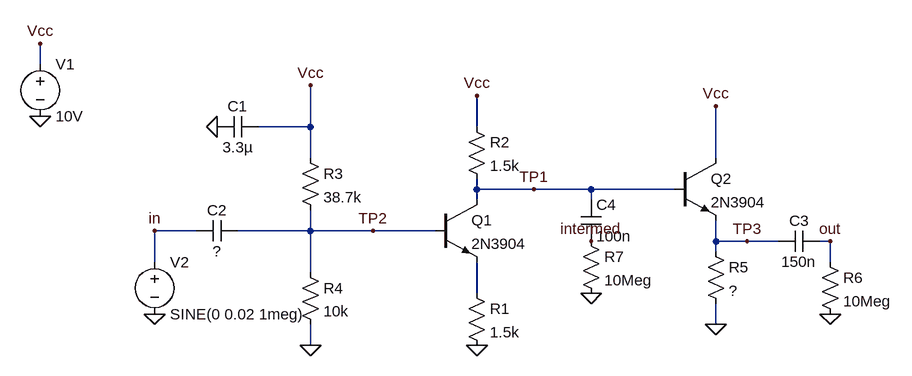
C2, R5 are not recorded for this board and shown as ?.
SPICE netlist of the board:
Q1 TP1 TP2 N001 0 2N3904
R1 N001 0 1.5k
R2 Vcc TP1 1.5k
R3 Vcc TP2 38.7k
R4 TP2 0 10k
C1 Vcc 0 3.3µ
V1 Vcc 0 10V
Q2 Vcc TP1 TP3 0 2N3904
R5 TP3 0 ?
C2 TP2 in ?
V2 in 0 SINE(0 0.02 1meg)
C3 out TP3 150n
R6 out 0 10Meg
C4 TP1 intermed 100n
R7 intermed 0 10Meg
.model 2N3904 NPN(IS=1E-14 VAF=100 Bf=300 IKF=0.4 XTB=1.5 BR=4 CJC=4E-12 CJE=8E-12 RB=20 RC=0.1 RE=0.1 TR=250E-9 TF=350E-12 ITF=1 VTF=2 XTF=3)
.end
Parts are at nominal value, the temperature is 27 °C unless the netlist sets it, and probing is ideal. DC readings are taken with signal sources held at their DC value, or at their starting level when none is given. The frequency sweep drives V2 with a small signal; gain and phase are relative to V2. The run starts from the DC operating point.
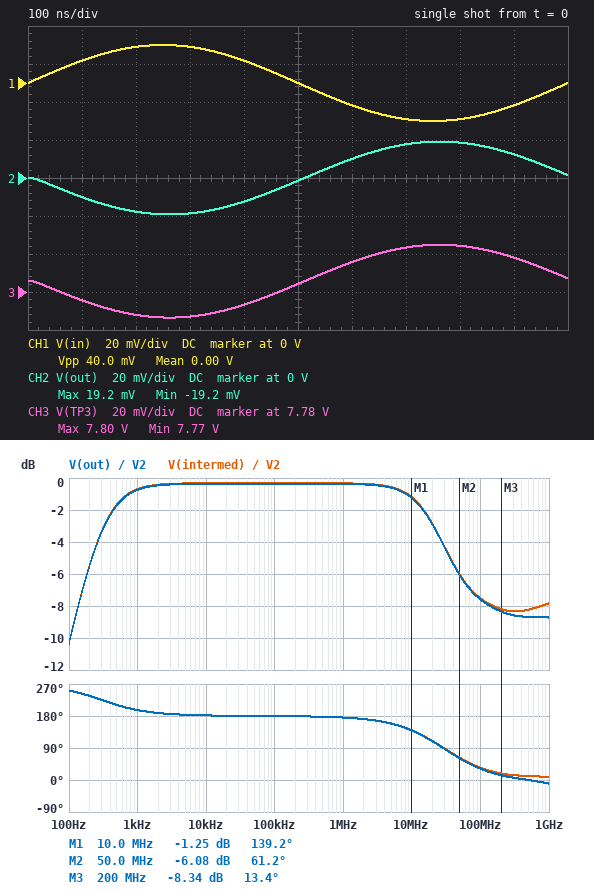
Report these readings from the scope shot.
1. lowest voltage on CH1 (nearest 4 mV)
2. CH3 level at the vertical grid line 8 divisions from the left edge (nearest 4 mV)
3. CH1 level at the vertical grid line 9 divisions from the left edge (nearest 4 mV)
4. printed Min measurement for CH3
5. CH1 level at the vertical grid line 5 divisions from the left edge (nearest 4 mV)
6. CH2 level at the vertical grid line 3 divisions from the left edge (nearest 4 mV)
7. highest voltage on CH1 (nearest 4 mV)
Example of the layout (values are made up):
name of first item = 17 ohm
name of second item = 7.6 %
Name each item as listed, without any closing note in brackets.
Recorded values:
lowest voltage on CH1 = -20 mV
CH3 level at the vertical grid line 8 divisions from the left edge = 7.804 V
CH1 level at the vertical grid line 9 divisions from the left edge = -12 mV
printed Min measurement for CH3 = 7.77 V
CH1 level at the vertical grid line 5 divisions from the left edge = 0 V
CH2 level at the vertical grid line 3 divisions from the left edge = -20 mV
highest voltage on CH1 = 20 mV
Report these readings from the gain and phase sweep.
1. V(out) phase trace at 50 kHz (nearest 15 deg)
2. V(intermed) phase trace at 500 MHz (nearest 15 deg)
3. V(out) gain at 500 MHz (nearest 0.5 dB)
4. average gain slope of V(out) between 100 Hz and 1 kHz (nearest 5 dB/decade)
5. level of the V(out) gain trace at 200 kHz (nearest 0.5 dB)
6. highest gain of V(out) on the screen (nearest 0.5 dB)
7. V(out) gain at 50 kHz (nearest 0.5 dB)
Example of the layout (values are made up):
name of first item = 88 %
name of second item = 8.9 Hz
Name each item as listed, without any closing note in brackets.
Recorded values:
V(out) phase trace at 50 kHz = 180 deg
V(intermed) phase trace at 500 MHz = 15 deg
V(out) gain at 500 MHz = -8.5 dB
average gain slope of V(out) between 100 Hz and 1 kHz = 10 dB/decade
level of the V(out) gain trace at 200 kHz = -0.5 dB
highest gain of V(out) on the screen = -0.5 dB
V(out) gain at 50 kHz = -0.5 dB
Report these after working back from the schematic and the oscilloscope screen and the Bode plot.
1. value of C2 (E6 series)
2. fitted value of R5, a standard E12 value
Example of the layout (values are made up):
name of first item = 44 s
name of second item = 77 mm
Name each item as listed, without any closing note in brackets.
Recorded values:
value of C2 = 68 nF
fitted value of R5, a standard E12 value = 390 Ω
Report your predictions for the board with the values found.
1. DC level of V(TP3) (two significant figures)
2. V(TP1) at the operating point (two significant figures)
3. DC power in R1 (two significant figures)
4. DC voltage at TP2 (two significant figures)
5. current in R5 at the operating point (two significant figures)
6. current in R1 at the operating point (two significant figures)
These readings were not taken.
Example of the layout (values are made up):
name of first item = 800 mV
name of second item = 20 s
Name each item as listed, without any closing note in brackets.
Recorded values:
DC level of V(TP3) = 7.8 V
V(TP1) at the operating point = 8.5 V
DC power in R1 = 1.3 mW
DC voltage at TP2 = 2.0 V
current in R5 at the operating point = 20 mA
current in R1 at the operating point = 920 µA
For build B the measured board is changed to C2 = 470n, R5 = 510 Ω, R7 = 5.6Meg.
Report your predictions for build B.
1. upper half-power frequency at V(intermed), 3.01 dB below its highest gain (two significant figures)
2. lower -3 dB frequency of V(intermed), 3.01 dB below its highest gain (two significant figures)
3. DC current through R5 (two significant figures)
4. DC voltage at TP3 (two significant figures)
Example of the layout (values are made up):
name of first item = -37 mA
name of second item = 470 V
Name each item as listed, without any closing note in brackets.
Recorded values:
upper half-power frequency at V(intermed), 3.01 dB below its highest gain = 24 MHz
lower -3 dB frequency of V(intermed), 3.01 dB below its highest gain = 43 Hz
DC current through R5 = 15 mA
DC voltage at TP3 = 7.8 V
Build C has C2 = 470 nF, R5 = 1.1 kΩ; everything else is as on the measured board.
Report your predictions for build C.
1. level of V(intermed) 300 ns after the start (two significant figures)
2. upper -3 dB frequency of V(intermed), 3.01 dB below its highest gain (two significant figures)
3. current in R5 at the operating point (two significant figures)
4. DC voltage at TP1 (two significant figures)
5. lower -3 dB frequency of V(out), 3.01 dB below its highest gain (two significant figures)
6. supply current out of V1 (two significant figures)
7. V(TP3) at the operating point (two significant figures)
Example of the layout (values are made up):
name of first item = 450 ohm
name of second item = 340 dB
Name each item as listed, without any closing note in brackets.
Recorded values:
level of V(intermed) 300 ns after the start = -19 mV
upper -3 dB frequency of V(intermed), 3.01 dB below its highest gain = 27 MHz
current in R5 at the operating point = 7.2 mA
DC voltage at TP1 = 8.6 V
lower -3 dB frequency of V(out), 3.01 dB below its highest gain = 43 Hz
supply current out of V1 = 8.3 mA
V(TP3) at the operating point = 7.9 V
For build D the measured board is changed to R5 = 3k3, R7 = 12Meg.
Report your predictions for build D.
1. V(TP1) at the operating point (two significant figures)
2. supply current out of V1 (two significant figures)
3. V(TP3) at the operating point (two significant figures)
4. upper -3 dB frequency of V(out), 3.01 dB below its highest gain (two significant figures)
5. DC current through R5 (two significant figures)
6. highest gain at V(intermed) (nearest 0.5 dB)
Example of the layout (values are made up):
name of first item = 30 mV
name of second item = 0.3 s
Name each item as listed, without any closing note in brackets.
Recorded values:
V(TP1) at the operating point = 8.6 V
supply current out of V1 = 3.5 mA
V(TP3) at the operating point = 7.9 V
upper -3 dB frequency of V(out), 3.01 dB below its highest gain = 29 MHz
DC current through R5 = 2.4 mA
highest gain at V(intermed) = 0 dB
